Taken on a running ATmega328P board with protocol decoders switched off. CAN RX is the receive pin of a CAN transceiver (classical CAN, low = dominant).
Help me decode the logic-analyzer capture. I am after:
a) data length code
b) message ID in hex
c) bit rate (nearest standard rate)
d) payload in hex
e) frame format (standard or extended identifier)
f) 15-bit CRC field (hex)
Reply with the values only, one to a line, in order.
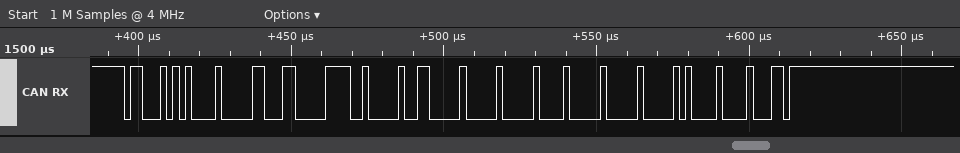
8
0x62A
500 kbit/s
23 07 20 30 00 01 00 00
standard
0x4211
